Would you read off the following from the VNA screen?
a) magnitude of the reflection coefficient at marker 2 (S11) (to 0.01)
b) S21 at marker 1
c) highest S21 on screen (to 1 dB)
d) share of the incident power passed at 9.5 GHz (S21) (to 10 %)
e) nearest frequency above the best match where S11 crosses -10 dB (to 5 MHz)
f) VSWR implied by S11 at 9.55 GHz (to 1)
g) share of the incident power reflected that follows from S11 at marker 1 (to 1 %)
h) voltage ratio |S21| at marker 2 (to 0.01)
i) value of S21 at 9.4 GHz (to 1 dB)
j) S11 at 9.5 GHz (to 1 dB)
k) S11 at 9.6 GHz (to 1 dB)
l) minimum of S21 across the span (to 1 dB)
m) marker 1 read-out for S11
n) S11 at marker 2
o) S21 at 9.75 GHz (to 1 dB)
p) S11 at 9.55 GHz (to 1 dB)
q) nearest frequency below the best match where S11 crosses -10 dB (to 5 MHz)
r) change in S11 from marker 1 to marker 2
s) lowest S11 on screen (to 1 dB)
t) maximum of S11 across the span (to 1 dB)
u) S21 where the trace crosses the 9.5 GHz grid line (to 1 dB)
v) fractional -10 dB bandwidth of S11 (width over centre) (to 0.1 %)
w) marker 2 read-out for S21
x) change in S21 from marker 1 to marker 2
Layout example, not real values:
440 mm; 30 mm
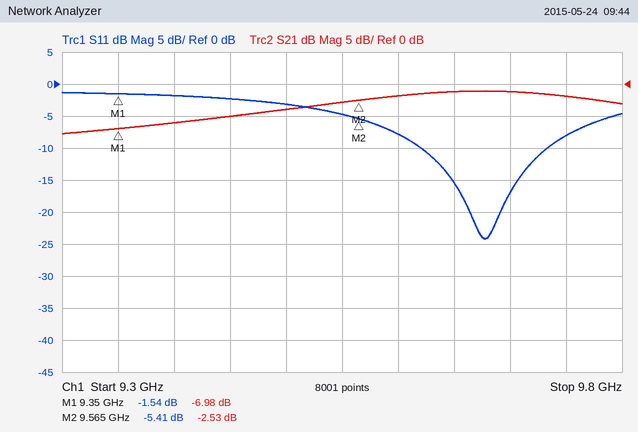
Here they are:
0.54; -6.98 dB; -1 dB; 40 %; 9.735 GHz; 4; 70 %; 0.75; -6 dB; -3 dB; -8 dB; -8 dB; -1.54 dB; -5.41 dB; -2 dB; -5 dB; 9.620 GHz; -3.87 dB; -24 dB; -1 dB; -4 dB; 1.2 %; -2.53 dB; 4.45 dB
